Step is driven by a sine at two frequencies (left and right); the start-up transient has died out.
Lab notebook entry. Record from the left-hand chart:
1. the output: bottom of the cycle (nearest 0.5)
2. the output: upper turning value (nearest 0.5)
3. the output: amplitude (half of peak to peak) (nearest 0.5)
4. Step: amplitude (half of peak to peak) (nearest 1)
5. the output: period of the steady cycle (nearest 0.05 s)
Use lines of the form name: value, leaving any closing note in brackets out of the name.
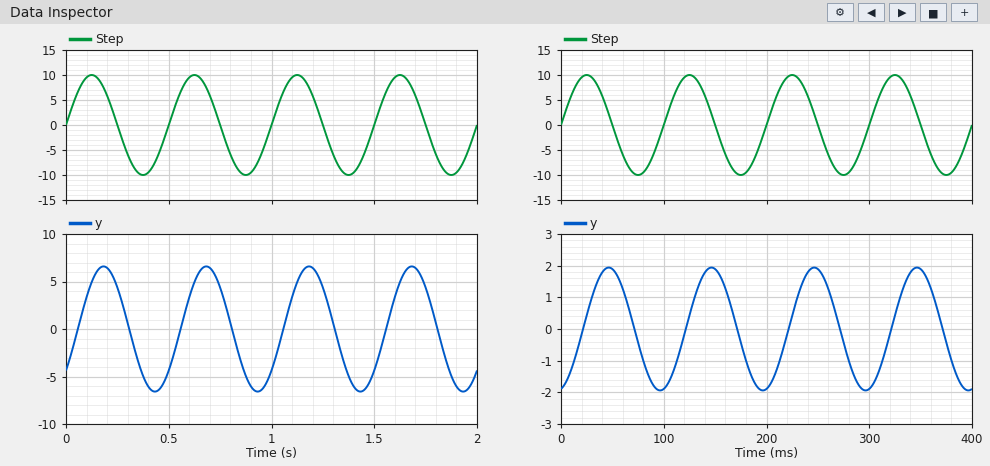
the output: bottom of the cycle: -6.5
the output: upper turning value: 6.5
the output: amplitude (half of peak to peak): 6.5
Step: amplitude (half of peak to peak): 10
the output: period of the steady cycle: 0.50 s
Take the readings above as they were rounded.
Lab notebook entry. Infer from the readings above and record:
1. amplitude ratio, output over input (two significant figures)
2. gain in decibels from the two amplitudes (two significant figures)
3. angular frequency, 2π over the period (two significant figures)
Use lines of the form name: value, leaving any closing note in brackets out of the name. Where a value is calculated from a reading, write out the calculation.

amplitude ratio, output over input: 6.5 / 10 = 0.65
gain in decibels from the two amplitudes: 20 log10(6.5 / 10) = -3.7 dB
angular frequency, 2π over the period: 2π / 0.5 = 13 rad/s
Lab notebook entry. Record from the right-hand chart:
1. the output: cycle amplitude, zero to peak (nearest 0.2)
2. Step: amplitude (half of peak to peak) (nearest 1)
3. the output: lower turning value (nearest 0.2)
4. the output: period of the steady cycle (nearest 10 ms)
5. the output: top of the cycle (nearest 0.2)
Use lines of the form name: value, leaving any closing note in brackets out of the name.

the output: cycle amplitude, zero to peak: 2.0
Step: amplitude (half of peak to peak): 10
the output: lower turning value: -2.0
the output: period of the steady cycle: 100 ms
the output: top of the cycle: 2.0
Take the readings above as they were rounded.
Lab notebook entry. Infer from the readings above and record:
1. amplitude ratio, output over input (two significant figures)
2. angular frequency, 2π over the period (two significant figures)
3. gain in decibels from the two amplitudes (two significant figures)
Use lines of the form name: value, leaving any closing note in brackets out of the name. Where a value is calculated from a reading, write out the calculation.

amplitude ratio, output over input: 2 / 10 = 0.20
angular frequency, 2π over the period: 2π / 100 = 0.063 rad/ms
gain in decibels from the two amplitudes: 20 log10(2 / 10) = -14 dB
